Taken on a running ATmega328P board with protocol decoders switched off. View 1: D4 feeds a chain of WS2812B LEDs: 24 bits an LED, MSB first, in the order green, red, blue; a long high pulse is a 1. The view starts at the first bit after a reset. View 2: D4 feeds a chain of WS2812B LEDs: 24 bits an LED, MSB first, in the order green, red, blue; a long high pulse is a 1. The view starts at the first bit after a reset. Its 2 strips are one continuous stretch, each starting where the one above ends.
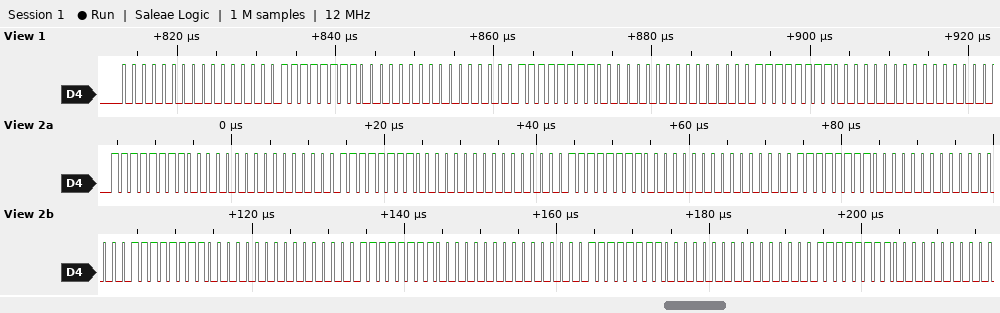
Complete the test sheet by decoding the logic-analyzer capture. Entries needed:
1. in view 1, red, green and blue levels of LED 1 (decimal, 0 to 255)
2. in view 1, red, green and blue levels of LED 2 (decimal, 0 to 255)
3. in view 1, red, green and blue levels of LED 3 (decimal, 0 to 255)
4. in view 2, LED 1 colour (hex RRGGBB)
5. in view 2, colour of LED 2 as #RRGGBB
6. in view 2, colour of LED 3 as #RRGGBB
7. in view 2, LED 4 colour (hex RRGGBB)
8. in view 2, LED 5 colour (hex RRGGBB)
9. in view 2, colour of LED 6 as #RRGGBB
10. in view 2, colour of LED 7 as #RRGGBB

0, 0, 255
0, 0, 255
0, 0, 255
#00FF00
#00FF00
#00FF00
#00FF00
#00FF00
#00FF00
#00FF00
